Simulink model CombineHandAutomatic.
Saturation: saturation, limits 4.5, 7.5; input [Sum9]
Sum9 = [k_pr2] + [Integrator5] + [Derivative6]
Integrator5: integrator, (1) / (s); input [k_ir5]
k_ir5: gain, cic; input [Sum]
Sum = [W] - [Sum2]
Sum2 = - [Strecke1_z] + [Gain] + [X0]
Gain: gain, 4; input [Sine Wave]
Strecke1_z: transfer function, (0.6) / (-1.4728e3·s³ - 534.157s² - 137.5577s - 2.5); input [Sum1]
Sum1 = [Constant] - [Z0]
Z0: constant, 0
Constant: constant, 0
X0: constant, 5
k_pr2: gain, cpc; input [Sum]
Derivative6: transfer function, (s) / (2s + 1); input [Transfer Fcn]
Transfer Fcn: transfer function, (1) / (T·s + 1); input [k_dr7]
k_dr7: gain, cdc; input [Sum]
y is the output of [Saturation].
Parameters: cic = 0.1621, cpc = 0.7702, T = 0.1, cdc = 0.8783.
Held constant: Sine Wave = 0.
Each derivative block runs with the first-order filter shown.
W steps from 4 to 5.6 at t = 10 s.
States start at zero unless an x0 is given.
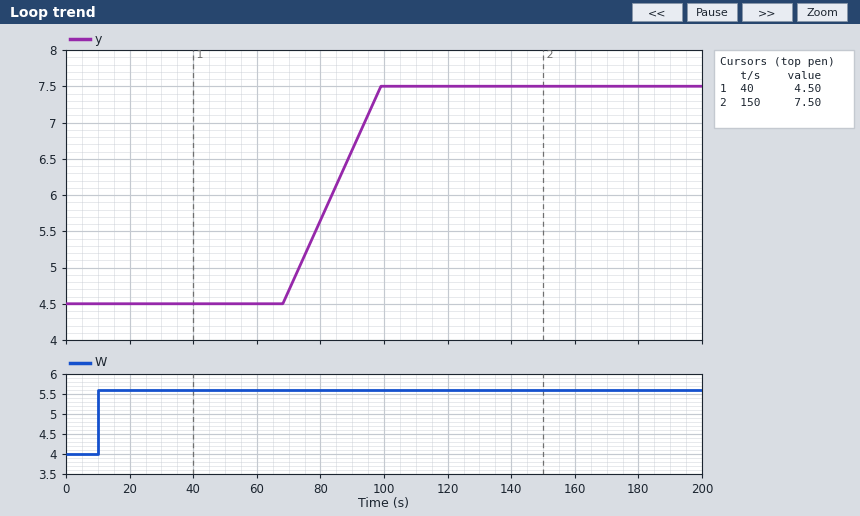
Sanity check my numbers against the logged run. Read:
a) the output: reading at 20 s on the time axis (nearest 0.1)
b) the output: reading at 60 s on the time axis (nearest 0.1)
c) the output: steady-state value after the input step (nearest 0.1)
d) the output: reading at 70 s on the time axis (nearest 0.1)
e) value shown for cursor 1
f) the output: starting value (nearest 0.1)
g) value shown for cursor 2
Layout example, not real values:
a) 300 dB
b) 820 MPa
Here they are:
a) 4.5
b) 4.5
c) 7.5
d) 4.7
e) 4.50
f) 4.5
g) 7.50
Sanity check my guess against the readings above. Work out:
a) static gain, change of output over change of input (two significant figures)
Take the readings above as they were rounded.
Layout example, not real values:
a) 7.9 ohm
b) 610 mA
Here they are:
a) 1.9
